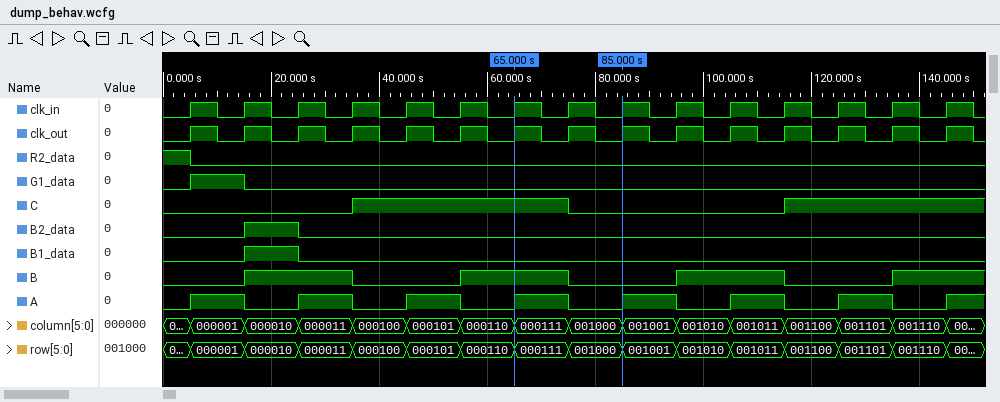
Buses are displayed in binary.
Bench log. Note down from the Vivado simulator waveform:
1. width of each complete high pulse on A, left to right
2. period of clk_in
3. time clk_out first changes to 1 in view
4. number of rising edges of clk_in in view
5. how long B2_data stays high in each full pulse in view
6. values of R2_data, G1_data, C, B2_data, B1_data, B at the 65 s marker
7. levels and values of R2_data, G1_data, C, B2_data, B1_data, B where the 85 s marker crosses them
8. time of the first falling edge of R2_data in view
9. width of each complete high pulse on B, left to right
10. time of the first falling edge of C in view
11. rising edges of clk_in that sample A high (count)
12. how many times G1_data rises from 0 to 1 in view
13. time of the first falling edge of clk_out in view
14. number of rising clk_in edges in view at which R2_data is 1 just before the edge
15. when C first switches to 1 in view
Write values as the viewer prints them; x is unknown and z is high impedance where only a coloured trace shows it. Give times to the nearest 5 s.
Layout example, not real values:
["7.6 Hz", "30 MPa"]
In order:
["10 s, 10 s, 10 s, 10 s, 10 s, 10 s, 10 s", "10 s", "5 s", "15", "10 s", "R2_data=0, G1_data=0, C=1, B2_data=0, B1_data=0, B=1", "R2_data=0, G1_data=0, C=0, B2_data=0, B1_data=0, B=0", "5 s", "20 s, 20 s, 20 s", "75 s", "7", "1", "10 s", "1", "35 s"]
